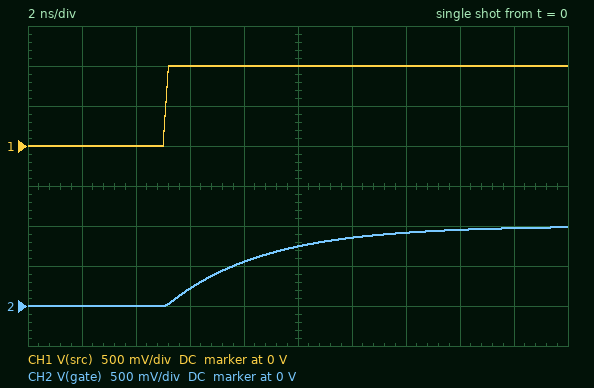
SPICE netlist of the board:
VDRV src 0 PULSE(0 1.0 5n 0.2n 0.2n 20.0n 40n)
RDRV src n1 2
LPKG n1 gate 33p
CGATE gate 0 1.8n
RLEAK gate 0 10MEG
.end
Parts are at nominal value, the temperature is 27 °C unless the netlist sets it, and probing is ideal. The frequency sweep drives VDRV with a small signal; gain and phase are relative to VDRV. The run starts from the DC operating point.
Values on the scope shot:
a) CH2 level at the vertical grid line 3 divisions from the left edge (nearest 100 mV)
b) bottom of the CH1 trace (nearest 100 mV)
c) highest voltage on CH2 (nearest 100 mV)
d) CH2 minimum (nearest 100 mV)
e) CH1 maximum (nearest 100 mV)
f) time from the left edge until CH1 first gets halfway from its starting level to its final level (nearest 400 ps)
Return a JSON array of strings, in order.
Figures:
["200 mV", "0 V", "1.0 V", "0 V", "1.0 V", "5.2 ns"]
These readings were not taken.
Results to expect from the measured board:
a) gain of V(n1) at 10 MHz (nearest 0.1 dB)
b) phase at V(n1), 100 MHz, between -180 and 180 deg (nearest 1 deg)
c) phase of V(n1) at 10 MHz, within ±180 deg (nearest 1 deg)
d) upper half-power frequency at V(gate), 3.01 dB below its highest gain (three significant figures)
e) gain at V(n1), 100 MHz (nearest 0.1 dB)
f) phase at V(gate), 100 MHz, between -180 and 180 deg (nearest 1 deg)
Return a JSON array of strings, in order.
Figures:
["-0.2 dB", "-67 deg", "-13 deg", "44.4 MHz", "-8.0 dB", "-67 deg"]
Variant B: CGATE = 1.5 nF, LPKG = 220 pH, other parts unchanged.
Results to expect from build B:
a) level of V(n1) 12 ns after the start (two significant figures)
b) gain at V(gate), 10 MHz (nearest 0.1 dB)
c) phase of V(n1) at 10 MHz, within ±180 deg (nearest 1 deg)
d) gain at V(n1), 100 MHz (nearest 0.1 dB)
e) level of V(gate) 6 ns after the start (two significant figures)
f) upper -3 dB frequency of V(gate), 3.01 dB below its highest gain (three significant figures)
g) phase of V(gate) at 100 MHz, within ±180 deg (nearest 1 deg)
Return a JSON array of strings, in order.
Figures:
["900 mV", "-0.1 dB", "-11 deg", "-7.6 dB", "240 mV", "55.1 MHz", "-65 deg"]
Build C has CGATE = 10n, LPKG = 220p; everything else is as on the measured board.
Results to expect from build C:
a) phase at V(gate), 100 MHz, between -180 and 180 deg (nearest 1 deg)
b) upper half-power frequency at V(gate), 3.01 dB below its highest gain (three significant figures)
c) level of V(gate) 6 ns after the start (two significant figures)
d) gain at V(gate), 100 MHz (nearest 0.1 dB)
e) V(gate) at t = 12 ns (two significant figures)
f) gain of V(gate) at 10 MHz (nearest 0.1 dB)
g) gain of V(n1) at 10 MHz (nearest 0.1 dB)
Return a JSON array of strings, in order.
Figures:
["-89 deg", "8.00 MHz", "39 mV", "-22.0 dB", "290 mV", "-4.1 dB", "-4.2 dB"]
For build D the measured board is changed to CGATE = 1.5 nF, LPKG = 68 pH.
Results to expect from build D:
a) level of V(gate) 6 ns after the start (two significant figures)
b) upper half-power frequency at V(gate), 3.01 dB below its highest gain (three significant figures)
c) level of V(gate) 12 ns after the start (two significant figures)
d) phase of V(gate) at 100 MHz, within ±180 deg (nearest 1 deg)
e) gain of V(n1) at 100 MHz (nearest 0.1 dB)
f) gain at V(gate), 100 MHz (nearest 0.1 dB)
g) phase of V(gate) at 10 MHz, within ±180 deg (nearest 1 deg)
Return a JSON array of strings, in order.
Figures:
["250 mV", "53.7 MHz", "900 mV", "-63 deg", "-6.9 dB", "-6.5 dB", "-11 deg"]
